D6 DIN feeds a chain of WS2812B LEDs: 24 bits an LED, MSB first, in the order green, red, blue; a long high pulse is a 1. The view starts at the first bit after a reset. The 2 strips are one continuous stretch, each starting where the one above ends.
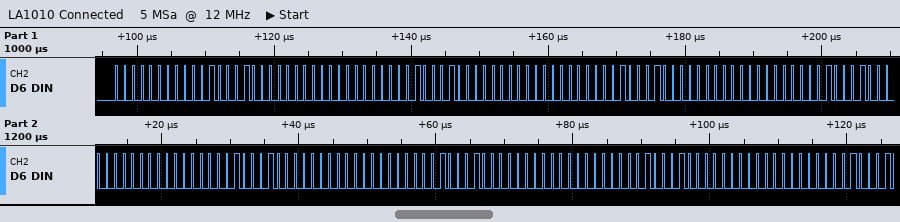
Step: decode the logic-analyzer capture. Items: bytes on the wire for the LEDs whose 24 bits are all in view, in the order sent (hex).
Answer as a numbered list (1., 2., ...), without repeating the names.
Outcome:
1. 00 11 00 00 11 00 00 11 00 00 11 00 00 11 00 00 11 00 00 11 00
